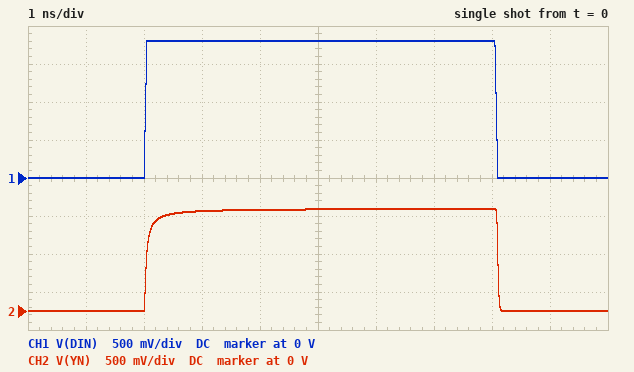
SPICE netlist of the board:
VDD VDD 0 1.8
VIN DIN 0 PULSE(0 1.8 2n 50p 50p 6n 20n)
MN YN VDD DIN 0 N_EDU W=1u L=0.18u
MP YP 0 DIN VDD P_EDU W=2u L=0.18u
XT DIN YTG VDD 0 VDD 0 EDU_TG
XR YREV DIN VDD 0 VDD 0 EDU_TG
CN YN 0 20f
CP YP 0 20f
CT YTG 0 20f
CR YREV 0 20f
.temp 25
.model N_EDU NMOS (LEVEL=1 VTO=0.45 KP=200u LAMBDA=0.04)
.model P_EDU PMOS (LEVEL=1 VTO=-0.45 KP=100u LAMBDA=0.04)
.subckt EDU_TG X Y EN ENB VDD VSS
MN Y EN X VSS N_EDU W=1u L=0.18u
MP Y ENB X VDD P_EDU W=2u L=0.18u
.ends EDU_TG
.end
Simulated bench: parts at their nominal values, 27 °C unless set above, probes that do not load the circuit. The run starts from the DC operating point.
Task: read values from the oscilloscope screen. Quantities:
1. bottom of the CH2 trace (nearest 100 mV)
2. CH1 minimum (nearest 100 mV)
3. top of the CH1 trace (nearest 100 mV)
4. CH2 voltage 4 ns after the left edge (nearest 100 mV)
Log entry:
0 V
0 V
1.8 V
1.3 V
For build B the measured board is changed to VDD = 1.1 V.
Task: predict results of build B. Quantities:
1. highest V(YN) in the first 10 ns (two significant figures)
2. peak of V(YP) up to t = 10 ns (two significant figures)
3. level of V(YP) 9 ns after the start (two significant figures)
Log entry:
640 mV
1.7 V
490 mV
